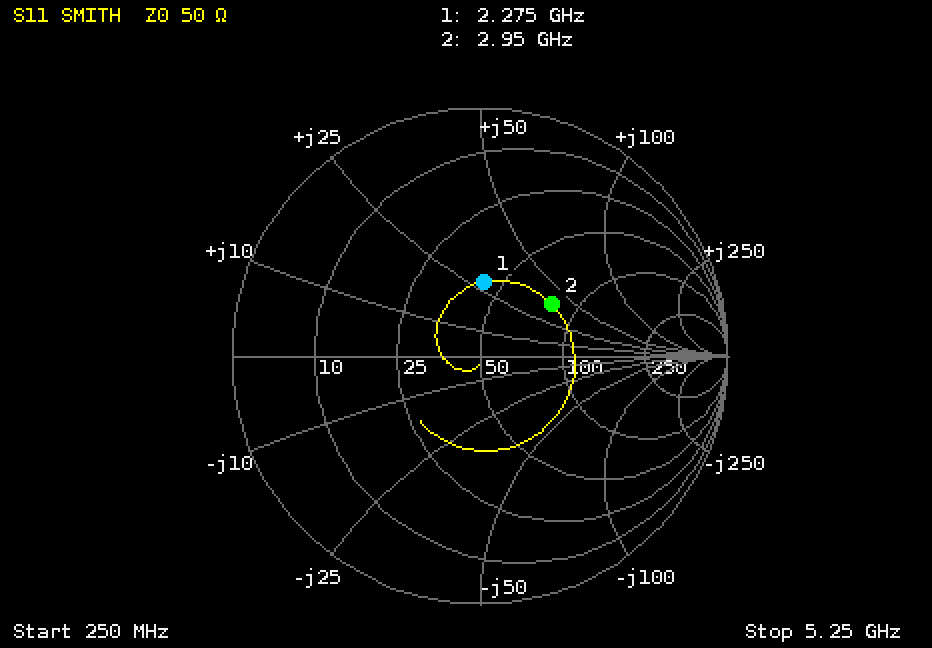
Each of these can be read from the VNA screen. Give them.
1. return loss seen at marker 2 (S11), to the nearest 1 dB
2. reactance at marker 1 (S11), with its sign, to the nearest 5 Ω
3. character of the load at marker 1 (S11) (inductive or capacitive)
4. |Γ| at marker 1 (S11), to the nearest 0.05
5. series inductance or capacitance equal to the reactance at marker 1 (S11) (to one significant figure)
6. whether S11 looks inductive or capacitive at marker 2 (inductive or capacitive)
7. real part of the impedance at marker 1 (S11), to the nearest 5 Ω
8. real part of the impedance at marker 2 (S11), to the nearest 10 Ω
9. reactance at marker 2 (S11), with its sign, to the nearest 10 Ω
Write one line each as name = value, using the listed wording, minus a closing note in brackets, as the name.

return loss seen at marker 2 (S11), to the nearest 1 dB = 9 dB
reactance at marker 1 (S11), with its sign, to the nearest 5 Ω = +30 Ω
character of the load at marker 1 (S11) = inductive
|Γ| at marker 1 (S11), to the nearest 0.05 = 0.30
series inductance or capacitance equal to the reactance at marker 1 (S11) = 2 nH
whether S11 looks inductive or capacitive at marker 2 = inductive
real part of the impedance at marker 1 (S11), to the nearest 5 Ω = 45 Ω
real part of the impedance at marker 2 (S11), to the nearest 10 Ω = 80 Ω
reactance at marker 2 (S11), with its sign, to the nearest 10 Ω = +40 Ω
